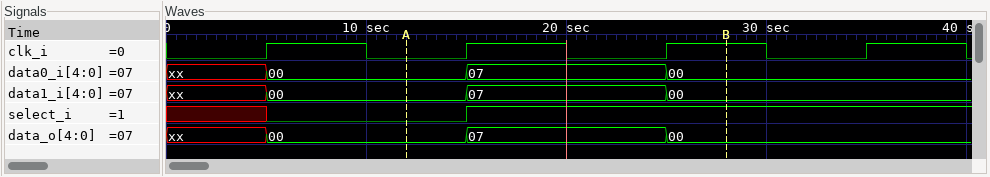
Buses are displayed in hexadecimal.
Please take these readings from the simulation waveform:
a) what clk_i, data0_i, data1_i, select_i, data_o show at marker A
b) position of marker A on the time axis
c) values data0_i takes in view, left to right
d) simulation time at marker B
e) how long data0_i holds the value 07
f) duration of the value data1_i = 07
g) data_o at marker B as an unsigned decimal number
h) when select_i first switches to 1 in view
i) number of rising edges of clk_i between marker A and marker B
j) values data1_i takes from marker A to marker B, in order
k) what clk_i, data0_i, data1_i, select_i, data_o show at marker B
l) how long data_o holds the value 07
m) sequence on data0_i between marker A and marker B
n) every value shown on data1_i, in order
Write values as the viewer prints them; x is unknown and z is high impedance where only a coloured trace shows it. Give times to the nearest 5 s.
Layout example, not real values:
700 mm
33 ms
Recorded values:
clk_i=0, data0_i=00, data1_i=00, select_i=0, data_o=00
10 s
xx, 00, 07, 00
30 s
10 s
10 s
0
15 s
2
00, 07, 00
clk_i=1, data0_i=00, data1_i=00, select_i=1, data_o=00
10 s
00, 07, 00
xx, 00, 07, 00
